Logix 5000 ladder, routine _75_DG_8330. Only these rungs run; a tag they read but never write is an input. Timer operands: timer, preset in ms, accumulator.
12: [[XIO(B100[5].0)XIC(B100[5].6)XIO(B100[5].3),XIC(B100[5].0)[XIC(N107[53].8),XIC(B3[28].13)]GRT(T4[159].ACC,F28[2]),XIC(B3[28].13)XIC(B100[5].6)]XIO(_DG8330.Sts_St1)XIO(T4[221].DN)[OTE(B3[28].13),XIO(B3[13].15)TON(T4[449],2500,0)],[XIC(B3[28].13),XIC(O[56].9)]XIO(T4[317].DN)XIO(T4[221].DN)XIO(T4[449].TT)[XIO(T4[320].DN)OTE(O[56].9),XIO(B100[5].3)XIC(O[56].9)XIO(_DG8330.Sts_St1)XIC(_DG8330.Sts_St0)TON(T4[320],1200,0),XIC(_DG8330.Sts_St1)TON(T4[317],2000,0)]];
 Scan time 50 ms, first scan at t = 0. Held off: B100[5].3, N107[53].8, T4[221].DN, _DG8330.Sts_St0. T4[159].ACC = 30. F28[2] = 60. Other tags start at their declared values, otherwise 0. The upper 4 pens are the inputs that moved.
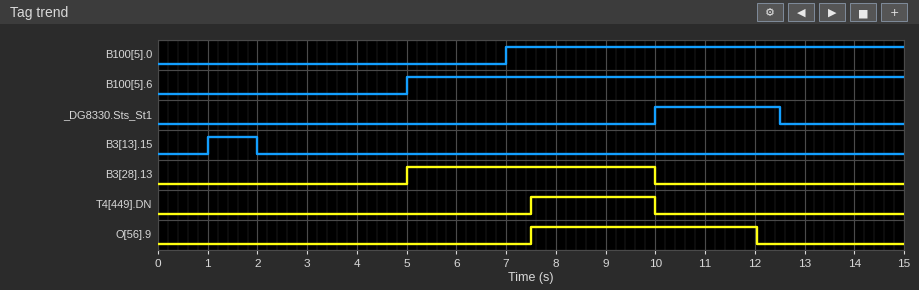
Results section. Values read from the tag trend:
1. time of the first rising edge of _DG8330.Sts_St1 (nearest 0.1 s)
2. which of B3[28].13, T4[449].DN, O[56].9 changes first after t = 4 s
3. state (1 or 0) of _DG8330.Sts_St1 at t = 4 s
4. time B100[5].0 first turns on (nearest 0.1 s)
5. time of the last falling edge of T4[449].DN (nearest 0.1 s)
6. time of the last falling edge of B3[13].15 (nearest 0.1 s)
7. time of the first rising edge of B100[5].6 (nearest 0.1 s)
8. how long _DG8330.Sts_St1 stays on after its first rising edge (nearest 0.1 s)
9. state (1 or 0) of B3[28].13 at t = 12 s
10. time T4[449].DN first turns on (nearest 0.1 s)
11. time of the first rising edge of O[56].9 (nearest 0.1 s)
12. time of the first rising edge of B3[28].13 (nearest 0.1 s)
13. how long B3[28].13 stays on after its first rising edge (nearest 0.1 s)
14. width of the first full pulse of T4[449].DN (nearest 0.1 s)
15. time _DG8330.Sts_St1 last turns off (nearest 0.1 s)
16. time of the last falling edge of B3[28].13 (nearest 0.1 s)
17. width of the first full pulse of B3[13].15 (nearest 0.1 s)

10.0 s
B3[28].13
0
7.0 s
10.0 s
2.0 s
5.0 s
2.5 s
0
7.5 s
7.5 s
5.0 s
5.0 s
2.5 s
12.5 s
10.0 s
1.0 s
